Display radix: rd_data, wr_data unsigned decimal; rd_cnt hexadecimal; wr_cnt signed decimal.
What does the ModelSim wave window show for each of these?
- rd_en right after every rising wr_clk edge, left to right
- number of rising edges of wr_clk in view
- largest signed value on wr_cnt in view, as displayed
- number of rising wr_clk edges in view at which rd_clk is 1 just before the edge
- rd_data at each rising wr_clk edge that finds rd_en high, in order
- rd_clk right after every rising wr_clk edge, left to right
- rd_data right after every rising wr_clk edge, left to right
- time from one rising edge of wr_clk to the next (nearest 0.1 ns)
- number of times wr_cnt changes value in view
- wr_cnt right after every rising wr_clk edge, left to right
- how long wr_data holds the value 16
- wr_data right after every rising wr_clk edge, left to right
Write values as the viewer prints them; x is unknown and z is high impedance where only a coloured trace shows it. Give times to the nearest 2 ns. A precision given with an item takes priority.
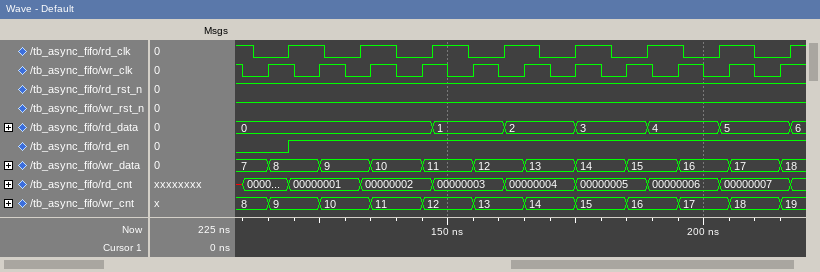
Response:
0 1 1 1 1 1 1 1 1 1 1
11
19
5
0, 0, 0, 1, 2, 2, 3, 4, 5, 5
0 1 1 0 0 1 1 0 1 1 0
0, 0, 0, 0, 1, 2, 3, 3, 4, 5, 5
10 ns
11
9, 10, 11, 12, 13, 14, 15, 16, 17, 18, 19
10 ns
8, 9, 10, 11, 12, 13, 14, 15, 16, 17, 18
